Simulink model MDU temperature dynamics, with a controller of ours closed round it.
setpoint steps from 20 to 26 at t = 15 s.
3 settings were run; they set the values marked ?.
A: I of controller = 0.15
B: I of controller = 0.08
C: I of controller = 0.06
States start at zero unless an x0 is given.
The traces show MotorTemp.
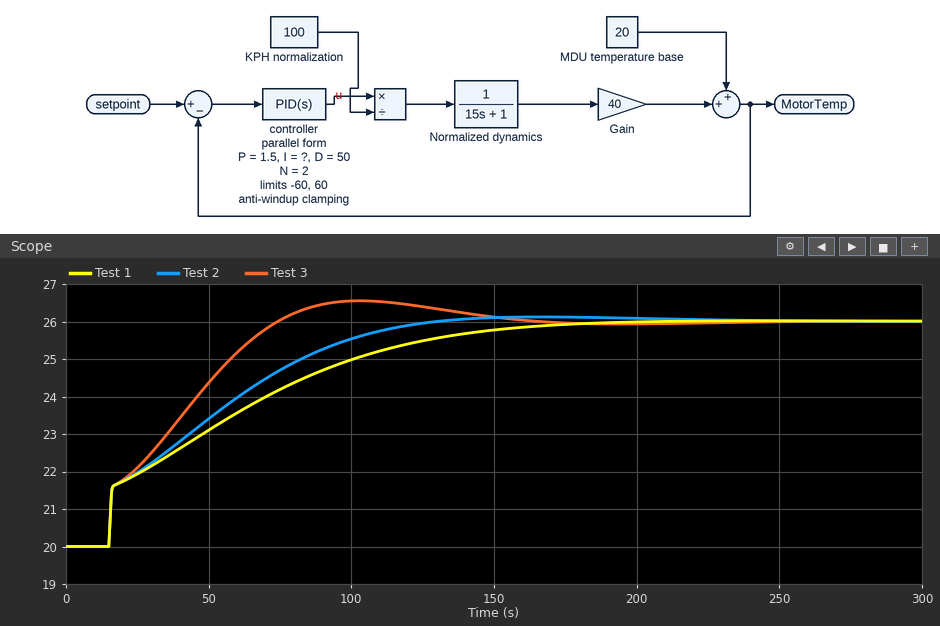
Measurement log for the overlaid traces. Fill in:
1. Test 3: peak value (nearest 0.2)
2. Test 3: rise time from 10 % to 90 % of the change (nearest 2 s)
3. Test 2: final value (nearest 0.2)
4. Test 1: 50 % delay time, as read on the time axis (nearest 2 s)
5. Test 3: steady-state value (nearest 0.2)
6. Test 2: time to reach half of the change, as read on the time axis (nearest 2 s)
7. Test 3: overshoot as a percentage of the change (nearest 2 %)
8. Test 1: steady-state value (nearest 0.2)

26.6
48 s
26.0
48 s
26.0
44 s
10 %
26.0
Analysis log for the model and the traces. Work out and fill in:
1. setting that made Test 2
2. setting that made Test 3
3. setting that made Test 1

B
A
C
